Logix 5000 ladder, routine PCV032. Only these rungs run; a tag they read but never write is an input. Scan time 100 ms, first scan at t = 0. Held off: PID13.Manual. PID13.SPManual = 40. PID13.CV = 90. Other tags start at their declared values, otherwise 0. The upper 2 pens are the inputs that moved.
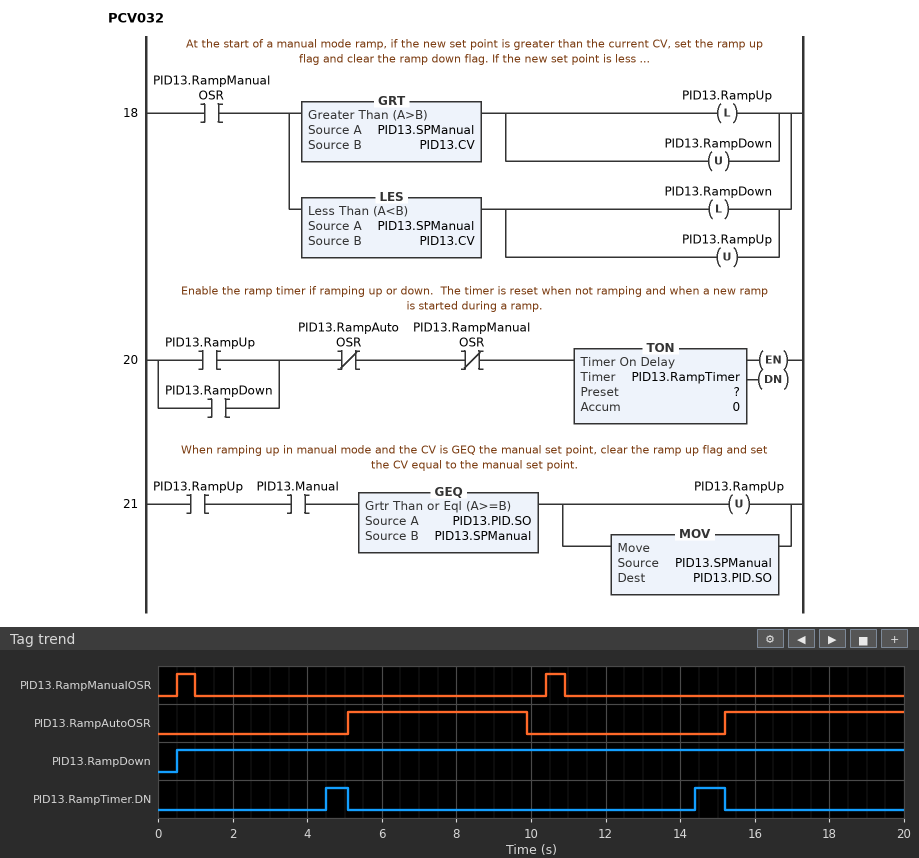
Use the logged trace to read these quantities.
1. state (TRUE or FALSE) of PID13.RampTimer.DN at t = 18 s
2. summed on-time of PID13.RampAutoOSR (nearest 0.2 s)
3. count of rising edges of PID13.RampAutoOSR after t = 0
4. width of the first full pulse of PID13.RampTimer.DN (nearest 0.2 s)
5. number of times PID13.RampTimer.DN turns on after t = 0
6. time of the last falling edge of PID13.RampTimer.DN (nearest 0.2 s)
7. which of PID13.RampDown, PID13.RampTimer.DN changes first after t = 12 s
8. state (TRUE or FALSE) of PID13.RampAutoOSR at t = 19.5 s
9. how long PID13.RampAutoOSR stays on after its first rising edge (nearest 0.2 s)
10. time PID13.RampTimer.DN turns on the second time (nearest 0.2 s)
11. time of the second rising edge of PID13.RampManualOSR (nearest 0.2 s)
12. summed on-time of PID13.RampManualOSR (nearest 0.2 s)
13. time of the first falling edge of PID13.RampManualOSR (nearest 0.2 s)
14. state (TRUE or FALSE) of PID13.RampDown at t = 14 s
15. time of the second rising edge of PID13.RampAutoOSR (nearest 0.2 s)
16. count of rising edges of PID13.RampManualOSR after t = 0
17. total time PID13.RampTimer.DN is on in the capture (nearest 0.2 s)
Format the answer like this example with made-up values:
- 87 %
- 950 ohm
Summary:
- FALSE
- 9.6 s
- 2
- 0.6 s
- 2
- 15.2 s
- PID13.RampTimer.DN
- TRUE
- 4.8 s
- 14.4 s
- 10.4 s
- 1.0 s
- 1.0 s
- TRUE
- 15.2 s
- 2
- 1.4 s
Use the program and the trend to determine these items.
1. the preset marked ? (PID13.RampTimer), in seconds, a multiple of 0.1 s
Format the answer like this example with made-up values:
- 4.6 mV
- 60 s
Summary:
- 3.5 s
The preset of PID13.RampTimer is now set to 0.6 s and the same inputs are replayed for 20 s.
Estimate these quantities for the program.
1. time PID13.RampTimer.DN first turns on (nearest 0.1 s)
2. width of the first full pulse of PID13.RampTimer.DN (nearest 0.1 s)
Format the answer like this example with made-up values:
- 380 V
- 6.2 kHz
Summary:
- 1.6 s
- 3.5 s
